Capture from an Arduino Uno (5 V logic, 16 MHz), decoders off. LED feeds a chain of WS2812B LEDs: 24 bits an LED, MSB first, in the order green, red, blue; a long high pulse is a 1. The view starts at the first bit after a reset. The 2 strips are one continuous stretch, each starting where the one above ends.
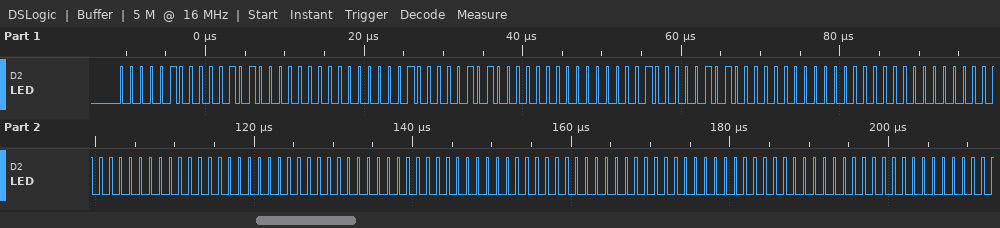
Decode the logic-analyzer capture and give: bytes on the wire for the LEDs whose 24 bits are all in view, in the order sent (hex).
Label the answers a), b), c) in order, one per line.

a) 04 14 00 04 14 00 04 14 00 00 00 00 00 00 00 00 00 00 00 00 00
